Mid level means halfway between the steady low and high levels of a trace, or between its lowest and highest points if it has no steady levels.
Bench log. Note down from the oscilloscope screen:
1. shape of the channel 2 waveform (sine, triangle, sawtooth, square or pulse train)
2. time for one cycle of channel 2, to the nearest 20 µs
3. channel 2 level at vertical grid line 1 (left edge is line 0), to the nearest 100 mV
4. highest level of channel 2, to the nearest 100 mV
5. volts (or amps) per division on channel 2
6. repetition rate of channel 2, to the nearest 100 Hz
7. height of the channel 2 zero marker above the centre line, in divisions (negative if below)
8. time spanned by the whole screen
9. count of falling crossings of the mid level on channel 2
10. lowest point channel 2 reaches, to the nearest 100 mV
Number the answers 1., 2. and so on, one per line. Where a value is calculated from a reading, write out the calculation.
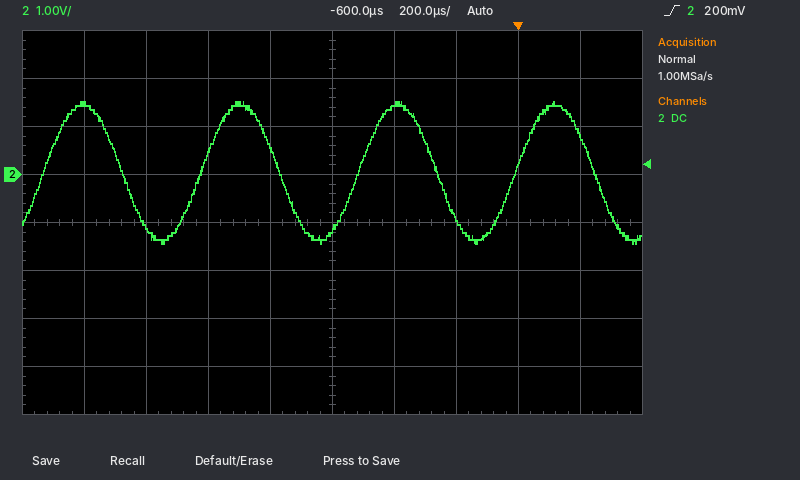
1. sine
2. 500 µs
3. 1.5 V
4. 1.5 V
5. 1 V
6. 1 / 500 µs ≈ 2.0 kHz
7. +1.0 div
8. 2 ms
9. 4
10. -1.4 V
